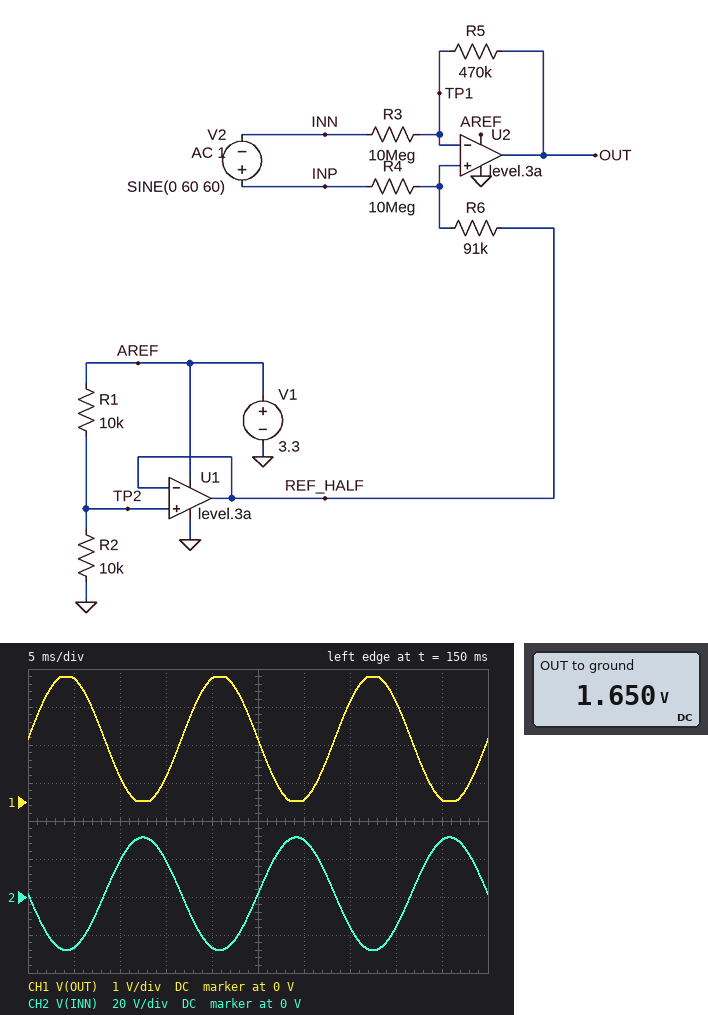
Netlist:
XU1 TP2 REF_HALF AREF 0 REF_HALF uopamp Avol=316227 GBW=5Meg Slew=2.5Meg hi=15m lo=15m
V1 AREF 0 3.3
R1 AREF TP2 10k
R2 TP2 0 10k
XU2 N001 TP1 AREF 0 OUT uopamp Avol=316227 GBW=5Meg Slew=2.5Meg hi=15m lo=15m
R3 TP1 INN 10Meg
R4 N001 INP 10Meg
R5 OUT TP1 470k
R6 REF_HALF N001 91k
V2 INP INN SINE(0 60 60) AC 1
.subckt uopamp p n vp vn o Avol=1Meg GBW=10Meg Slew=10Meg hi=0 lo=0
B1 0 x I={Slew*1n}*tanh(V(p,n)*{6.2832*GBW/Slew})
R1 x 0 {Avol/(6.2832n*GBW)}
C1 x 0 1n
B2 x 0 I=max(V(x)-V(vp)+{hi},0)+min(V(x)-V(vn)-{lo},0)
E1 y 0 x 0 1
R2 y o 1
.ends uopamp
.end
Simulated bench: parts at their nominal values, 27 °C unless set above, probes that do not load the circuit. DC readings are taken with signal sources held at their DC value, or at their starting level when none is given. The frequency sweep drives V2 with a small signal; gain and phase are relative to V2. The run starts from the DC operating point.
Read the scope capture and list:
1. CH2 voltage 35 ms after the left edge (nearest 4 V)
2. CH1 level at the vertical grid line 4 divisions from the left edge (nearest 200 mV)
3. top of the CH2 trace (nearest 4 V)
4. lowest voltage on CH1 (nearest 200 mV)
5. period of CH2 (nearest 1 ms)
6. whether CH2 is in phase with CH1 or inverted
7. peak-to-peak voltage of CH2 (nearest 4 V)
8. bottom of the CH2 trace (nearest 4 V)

-16 V
3.2 V
32 V
0 V
17 ms
inverted
60 V
-28 V
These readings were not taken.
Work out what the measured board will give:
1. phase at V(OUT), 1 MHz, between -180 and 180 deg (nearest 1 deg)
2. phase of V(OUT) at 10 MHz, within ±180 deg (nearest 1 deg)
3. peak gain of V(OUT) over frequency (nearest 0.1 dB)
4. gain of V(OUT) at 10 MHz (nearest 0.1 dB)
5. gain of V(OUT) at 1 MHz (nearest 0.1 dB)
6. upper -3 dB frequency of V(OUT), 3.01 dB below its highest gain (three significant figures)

-12 deg
-64 deg
-31.0 dB
-38.2 dB
-31.2 dB
4.86 MHz
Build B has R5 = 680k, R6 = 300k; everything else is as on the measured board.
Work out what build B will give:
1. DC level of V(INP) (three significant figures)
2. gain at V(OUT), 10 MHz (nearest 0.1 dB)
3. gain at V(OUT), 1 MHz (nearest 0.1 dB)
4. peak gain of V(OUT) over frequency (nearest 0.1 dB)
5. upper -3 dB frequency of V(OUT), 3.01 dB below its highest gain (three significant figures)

1.65 V
-33.5 dB
-26.4 dB
-26.2 dB
4.77 MHz
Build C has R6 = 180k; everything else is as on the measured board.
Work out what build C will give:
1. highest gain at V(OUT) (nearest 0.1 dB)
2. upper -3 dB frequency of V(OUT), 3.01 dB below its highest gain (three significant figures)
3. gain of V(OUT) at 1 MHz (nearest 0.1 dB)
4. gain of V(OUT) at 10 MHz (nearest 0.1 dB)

-29.8 dB
4.84 MHz
-29.9 dB
-37.0 dB
